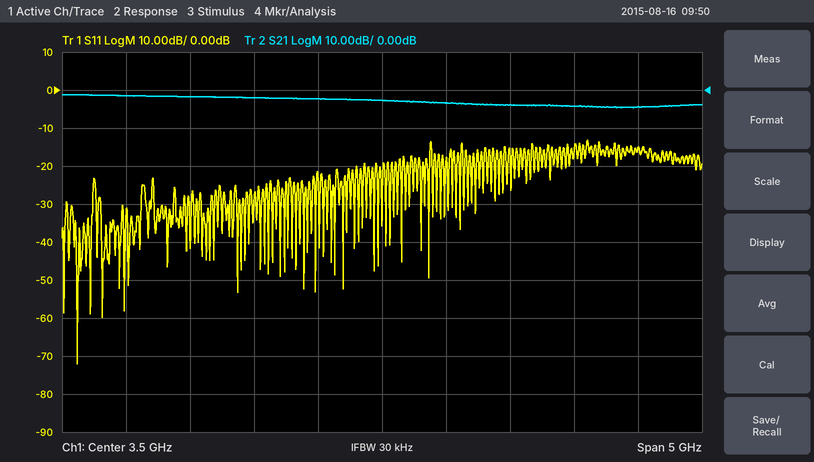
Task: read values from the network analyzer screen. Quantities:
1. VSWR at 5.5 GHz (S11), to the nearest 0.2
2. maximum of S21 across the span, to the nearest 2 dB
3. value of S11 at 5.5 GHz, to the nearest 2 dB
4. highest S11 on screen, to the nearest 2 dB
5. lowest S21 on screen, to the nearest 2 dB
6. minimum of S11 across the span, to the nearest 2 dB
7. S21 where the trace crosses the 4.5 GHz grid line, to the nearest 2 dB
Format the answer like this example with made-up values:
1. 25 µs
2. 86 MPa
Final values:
1. 1.4
2. -2 dB
3. -16 dB
4. -14 dB
5. -4 dB
6. -72 dB
7. -4 dB
